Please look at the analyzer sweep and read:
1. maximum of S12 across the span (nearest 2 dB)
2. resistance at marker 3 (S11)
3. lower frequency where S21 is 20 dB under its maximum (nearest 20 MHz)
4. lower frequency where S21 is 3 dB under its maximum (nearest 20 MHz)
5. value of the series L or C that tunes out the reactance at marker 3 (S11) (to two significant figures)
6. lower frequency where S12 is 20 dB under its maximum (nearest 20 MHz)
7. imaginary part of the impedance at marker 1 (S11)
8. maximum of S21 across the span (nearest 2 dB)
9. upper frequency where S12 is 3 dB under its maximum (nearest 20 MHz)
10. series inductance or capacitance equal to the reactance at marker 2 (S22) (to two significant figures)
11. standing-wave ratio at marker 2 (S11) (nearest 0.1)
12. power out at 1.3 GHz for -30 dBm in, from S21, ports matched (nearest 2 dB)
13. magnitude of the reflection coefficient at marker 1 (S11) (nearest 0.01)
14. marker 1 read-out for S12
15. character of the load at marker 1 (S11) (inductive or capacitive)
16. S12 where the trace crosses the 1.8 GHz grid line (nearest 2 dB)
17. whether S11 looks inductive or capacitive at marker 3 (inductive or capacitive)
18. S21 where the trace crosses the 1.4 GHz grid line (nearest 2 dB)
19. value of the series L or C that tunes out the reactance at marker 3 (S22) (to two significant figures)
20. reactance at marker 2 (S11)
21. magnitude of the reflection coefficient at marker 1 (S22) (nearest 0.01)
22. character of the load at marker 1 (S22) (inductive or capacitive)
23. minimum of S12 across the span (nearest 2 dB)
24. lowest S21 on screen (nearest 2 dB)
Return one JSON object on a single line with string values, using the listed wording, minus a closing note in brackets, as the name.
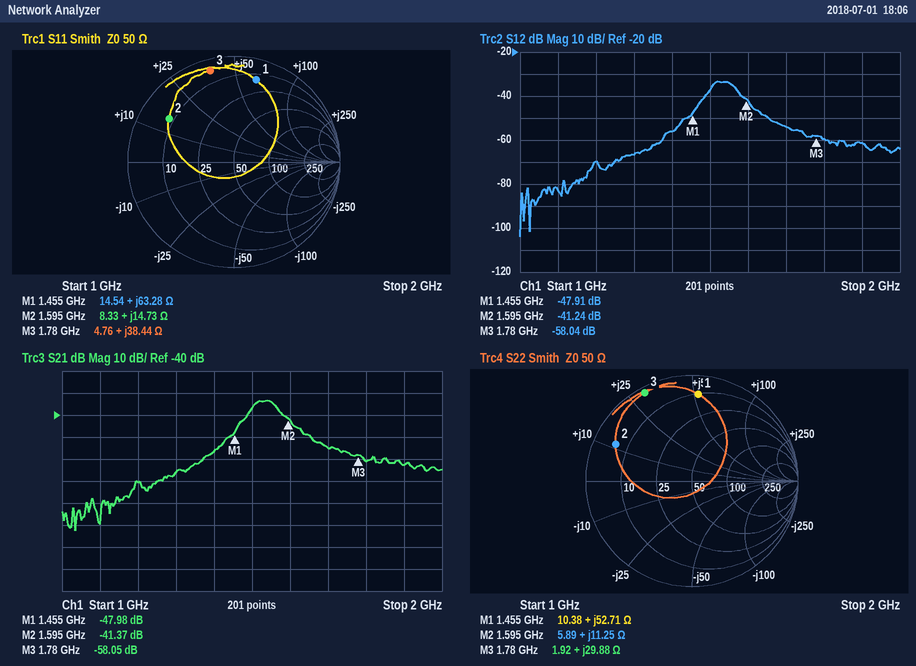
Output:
{"maximum of S12 across the span": "-34 dB", "resistance at marker 3": "4.76 Ω", "lower frequency where S21 is 20 dB under its maximum": "1.42 GHz", "lower frequency where S21 is 3 dB under its maximum": "1.50 GHz", "value of the series L or C that tunes out the reactance at marker 3 (S11)": "2.3 pF", "lower frequency where S12 is 20 dB under its maximum": "1.42 GHz", "imaginary part of the impedance at marker 1": "+63.28 Ω", "maximum of S21 across the span": "-34 dB", "upper frequency where S12 is 3 dB under its maximum": "1.56 GHz", "series inductance or capacitance equal to the reactance at marker 2 (S22)": "1.1 nH", "standing-wave ratio at marker 2 (S11)": "6.5", "power out at 1.3 GHz for -30 dBm in, from S21, ports matched": "-96 dBm", "magnitude of the reflection coefficient at marker 1 (S11)": "0.80", "marker 1 read-out for S12": "-47.91 dB", "character of the load at marker 1 (S11)": "inductive", "S12 where the trace crosses the 1.8 GHz grid line": "-60 dB", "whether S11 looks inductive or capacitive at marker 3": "inductive", "S21 where the trace crosses the 1.4 GHz grid line": "-56 dB", "value of the series L or C that tunes out the reactance at marker 3 (S22)": "3.0 pF", "reactance at marker 2": "+14.73 Ω", "magnitude of the reflection coefficient at marker 1 (S22)": "0.82", "character of the load at marker 1 (S22)": "inductive", "minimum of S12 across the span": "-104 dB", "lowest S21 on screen": "-92 dB"}
